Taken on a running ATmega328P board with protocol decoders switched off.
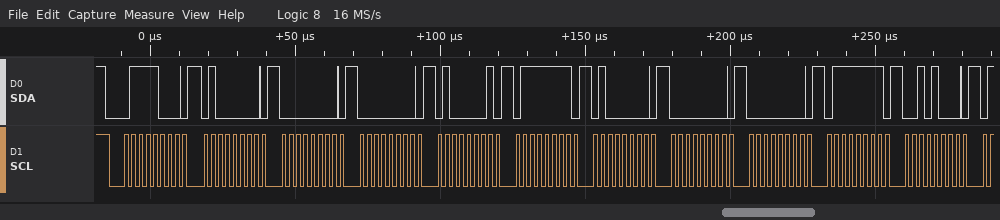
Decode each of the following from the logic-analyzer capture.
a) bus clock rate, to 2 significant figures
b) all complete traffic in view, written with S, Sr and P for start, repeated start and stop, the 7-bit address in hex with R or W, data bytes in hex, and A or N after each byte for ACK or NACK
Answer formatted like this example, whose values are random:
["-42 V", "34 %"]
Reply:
["400 kHz", "S 3CW A 40 A 00 A 00 A 41 A 7F A 40 A 00 A 00 A 7F A 28 A"]
